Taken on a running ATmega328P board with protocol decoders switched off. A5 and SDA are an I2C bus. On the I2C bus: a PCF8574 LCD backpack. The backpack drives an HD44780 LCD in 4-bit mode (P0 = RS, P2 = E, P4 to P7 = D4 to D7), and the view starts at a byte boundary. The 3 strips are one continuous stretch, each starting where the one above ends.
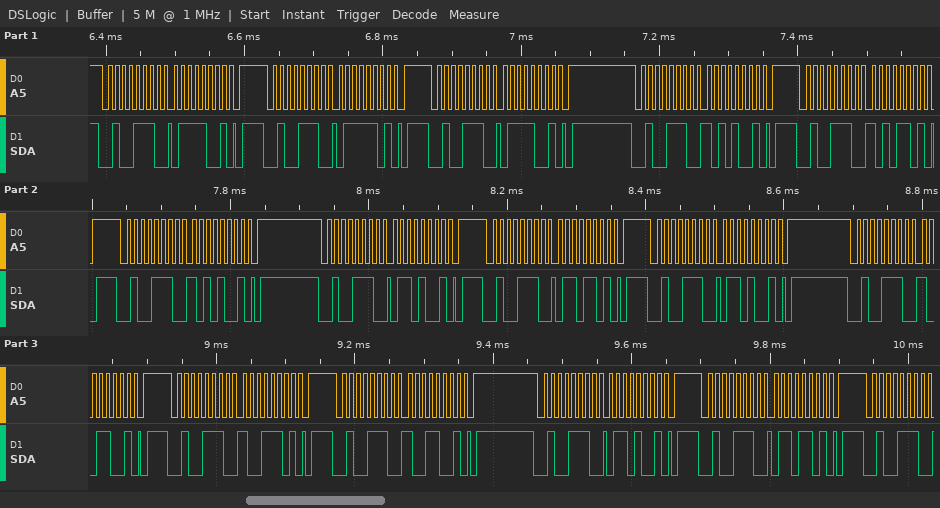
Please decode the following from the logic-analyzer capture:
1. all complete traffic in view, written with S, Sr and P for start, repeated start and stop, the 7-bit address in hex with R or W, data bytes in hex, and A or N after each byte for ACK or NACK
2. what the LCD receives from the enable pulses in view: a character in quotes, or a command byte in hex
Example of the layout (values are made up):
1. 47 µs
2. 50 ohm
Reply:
1. S 27W A 79 A P S 27W A 7D A P S 27W A 79 A P S 27W A A9 A P S 27W A AD A P S 27W A A9 A P S 27W A 69 A P S 27W A 6D A P S 27W A 69 A P S 27W A 99 A P S 27W A 9D A P S 27W A 99 A P S 27W A 69 A P S 27W A 6D A P S 27W A
2. 'z' 'i'
